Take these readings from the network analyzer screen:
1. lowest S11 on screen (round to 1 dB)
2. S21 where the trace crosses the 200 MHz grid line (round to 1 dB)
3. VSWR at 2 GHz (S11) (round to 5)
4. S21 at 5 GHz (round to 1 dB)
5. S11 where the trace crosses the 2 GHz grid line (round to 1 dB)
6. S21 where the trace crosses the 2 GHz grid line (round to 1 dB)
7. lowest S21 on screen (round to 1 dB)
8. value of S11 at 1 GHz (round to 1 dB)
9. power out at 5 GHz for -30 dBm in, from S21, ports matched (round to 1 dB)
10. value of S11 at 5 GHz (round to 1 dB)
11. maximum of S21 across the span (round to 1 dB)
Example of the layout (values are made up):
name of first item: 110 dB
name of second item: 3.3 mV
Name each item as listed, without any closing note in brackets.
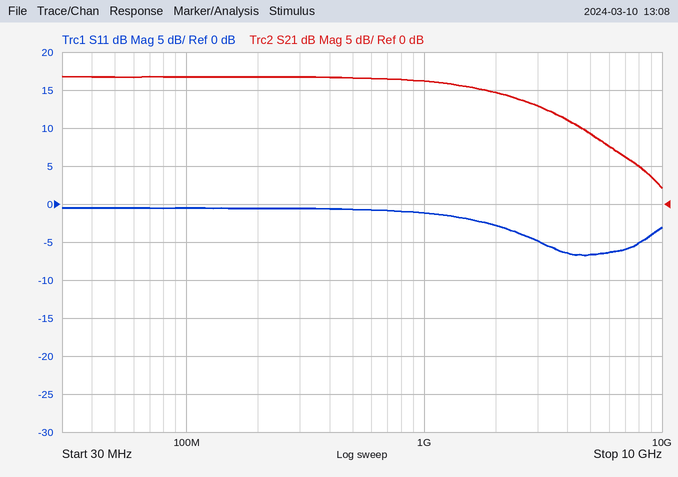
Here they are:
lowest S11 on screen: -7 dB
S21 where the trace crosses the 200 MHz grid line: 17 dB
VSWR at 2 GHz (S11): 5
S21 at 5 GHz: 9 dB
S11 where the trace crosses the 2 GHz grid line: -3 dB
S21 where the trace crosses the 2 GHz grid line: 15 dB
lowest S21 on screen: 2 dB
value of S11 at 1 GHz: -1 dB
power out at 5 GHz for -30 dBm in, from S21, ports matched: -21 dBm
value of S11 at 5 GHz: -7 dB
maximum of S21 across the span: 17 dB
